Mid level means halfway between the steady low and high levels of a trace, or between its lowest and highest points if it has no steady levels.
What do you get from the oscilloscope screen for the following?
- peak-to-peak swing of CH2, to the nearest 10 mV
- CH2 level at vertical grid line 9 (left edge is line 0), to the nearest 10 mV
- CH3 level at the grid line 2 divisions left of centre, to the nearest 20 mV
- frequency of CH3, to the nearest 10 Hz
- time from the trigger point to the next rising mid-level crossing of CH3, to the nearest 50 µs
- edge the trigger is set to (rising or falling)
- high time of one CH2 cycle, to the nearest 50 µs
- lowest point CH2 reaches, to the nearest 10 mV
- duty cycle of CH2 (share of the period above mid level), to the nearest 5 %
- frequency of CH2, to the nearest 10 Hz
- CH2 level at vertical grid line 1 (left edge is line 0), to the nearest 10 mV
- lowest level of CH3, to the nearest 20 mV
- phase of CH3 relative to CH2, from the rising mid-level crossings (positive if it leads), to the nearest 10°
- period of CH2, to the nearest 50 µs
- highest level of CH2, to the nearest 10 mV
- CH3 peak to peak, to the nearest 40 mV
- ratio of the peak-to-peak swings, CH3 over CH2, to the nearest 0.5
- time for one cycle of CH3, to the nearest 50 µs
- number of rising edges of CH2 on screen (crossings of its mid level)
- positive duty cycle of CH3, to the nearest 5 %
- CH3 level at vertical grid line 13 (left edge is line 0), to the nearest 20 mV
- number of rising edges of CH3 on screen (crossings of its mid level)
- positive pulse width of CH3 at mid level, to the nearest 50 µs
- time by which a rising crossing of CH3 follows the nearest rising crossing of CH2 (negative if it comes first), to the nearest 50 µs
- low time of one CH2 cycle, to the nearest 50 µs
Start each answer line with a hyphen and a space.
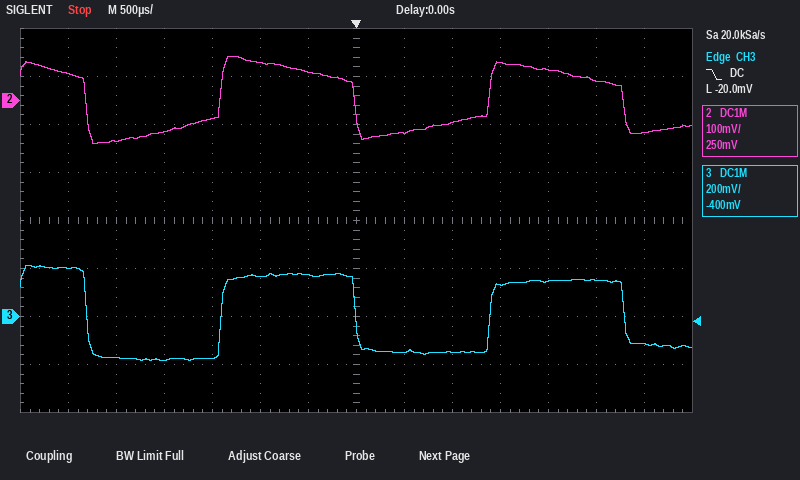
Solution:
- 180 mV
- -50 mV
- 160 mV
- 360 Hz
- 1.40 ms
- falling
- 1.40 ms
- -90 mV
- 50 %
- 360 Hz
- 60 mV
- -180 mV
- 0°
- 2.80 ms
- 90 mV
- 400 mV
- 2.0
- 2.80 ms
- 2
- 50 %
- -120 mV
- 2
- 1.40 ms
- 0 µs
- 1.40 ms
